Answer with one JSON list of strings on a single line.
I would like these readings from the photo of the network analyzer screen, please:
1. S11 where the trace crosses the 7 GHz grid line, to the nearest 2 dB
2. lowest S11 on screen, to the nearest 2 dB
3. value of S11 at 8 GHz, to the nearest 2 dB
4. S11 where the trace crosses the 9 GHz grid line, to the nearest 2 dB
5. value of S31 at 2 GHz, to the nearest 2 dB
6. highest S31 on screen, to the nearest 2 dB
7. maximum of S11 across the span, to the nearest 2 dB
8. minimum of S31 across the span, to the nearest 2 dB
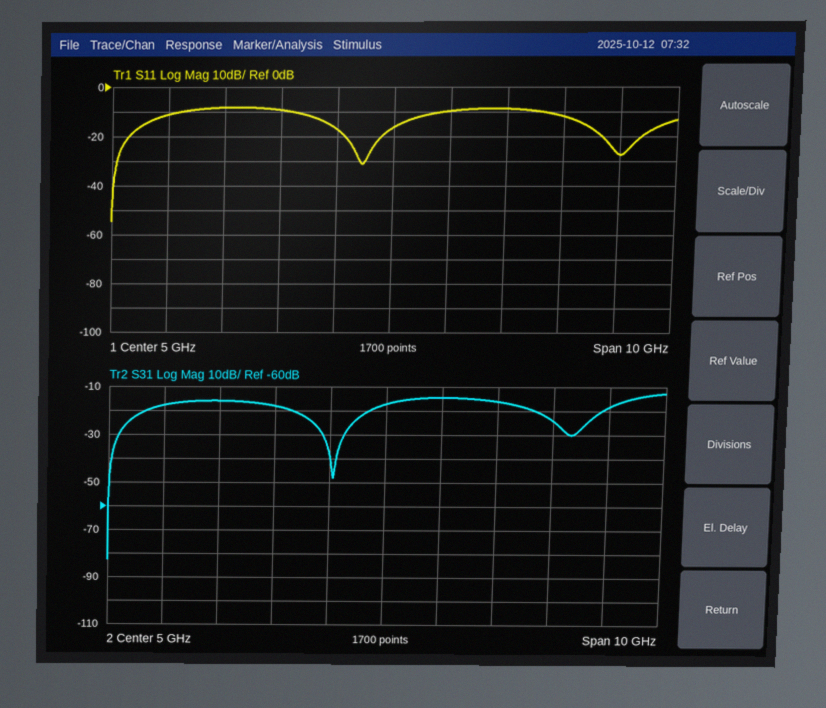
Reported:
["-8 dB", "-54 dB", "-12 dB", "-28 dB", "-16 dB", "-12 dB", "-8 dB", "-82 dB"]
